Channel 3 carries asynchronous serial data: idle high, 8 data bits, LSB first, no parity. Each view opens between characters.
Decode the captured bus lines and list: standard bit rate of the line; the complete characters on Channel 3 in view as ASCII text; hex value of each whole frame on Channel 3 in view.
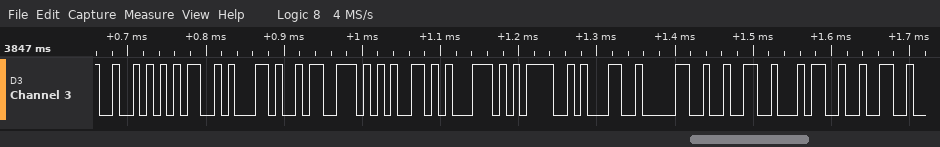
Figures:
115200 baud
"RM,seq=10242"
52, 4D, 2C, 73, 65, 71, 3D, 31, 30, 32, 34, 32
